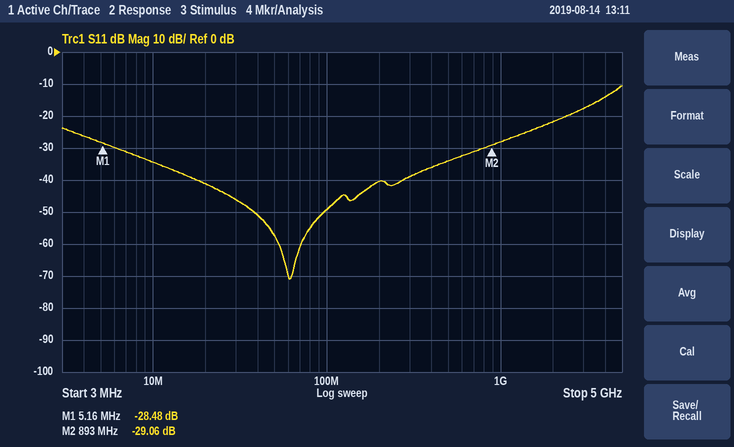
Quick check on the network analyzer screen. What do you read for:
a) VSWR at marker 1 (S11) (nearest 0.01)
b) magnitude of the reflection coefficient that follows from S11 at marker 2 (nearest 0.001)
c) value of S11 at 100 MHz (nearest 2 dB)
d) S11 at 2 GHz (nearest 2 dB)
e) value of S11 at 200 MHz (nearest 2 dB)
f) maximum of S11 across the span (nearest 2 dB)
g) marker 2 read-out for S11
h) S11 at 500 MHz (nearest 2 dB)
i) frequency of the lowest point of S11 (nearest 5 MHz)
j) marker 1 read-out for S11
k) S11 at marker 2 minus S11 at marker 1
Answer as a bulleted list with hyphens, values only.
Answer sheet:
- 1.08
- 0.035
- -50 dB
- -22 dB
- -40 dB
- -10 dB
- -29.06 dB
- -34 dB
- 60 MHz
- -28.48 dB
- -0.58 dB
